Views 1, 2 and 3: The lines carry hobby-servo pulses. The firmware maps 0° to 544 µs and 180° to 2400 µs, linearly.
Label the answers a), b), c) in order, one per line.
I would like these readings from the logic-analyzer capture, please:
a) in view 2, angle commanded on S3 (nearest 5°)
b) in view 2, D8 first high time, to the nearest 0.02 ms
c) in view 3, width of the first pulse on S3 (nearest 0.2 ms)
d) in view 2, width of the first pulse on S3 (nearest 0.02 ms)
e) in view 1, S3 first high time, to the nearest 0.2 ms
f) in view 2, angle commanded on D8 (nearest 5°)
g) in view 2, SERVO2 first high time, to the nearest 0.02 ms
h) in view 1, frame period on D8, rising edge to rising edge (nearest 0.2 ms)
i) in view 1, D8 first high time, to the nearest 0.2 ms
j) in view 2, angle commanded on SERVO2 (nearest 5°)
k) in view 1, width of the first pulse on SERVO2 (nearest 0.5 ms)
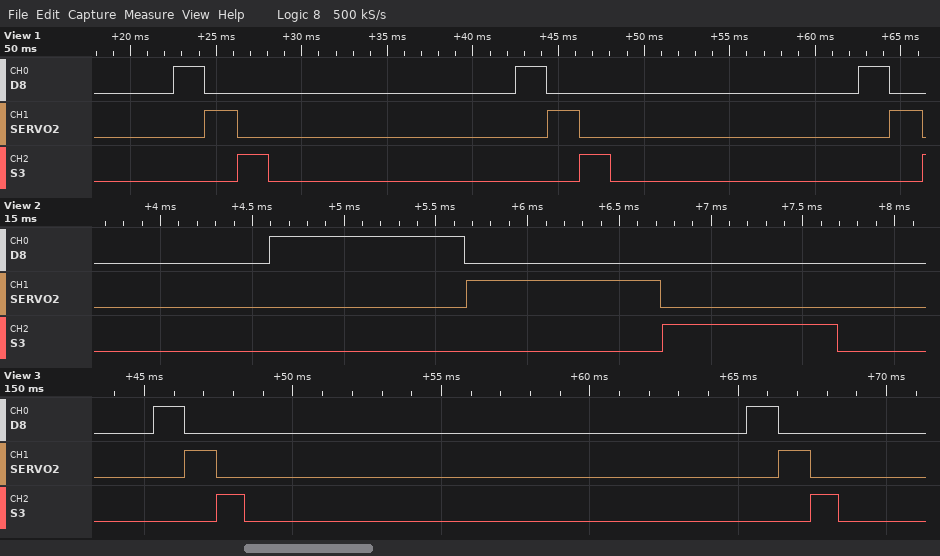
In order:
a) 40°
b) 1.06 ms
c) 1.0 ms
d) 0.96 ms
e) 1.8 ms
f) 50°
g) 1.06 ms
h) 20.0 ms
i) 1.8 ms
j) 50°
k) 2.0 ms
